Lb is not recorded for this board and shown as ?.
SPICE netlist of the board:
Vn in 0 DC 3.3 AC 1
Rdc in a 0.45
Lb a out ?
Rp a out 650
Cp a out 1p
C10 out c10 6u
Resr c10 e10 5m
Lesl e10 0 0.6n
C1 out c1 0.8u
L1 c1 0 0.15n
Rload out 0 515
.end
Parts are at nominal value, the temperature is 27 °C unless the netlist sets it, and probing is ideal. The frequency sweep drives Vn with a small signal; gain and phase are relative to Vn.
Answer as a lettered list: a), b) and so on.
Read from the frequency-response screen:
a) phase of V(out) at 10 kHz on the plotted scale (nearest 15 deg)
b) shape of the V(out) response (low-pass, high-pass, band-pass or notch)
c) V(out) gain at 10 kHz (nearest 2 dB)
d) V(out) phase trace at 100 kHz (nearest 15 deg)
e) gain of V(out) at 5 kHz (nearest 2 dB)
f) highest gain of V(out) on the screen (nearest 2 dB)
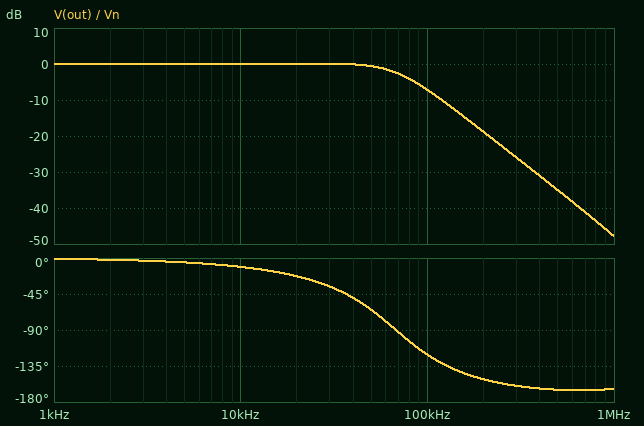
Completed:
a) -15 deg
b) low-pass
c) 0 dB
d) -120 deg
e) 0 dB
f) 0 dB
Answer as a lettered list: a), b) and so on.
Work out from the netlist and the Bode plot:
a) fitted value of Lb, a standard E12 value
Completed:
a) 820 nH
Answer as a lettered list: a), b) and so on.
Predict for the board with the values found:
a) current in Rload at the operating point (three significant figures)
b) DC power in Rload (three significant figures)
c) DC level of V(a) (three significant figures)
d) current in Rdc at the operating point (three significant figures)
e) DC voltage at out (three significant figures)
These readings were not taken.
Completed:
a) 6.40 mA
b) 21.1 mW
c) 3.30 V
d) 6.40 mA
e) 3.30 V
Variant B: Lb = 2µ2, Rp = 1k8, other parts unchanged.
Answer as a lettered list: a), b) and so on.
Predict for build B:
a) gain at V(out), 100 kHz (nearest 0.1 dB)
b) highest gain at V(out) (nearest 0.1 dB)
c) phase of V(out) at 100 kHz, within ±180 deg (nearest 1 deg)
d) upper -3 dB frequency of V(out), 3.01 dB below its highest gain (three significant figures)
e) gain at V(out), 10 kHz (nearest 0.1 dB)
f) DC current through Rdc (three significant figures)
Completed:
a) -14.5 dB
b) 2.7 dB
c) -157 deg
d) 48.9 kHz
e) 0.3 dB
f) 6.40 mA
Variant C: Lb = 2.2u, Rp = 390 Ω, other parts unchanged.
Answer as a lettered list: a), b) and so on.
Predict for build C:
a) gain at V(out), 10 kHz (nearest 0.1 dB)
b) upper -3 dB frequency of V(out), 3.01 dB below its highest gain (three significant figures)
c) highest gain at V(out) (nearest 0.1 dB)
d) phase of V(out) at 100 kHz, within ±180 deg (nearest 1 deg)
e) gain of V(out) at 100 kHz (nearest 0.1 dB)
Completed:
a) 0.3 dB
b) 48.9 kHz
c) 2.7 dB
d) -157 deg
e) -14.5 dB
